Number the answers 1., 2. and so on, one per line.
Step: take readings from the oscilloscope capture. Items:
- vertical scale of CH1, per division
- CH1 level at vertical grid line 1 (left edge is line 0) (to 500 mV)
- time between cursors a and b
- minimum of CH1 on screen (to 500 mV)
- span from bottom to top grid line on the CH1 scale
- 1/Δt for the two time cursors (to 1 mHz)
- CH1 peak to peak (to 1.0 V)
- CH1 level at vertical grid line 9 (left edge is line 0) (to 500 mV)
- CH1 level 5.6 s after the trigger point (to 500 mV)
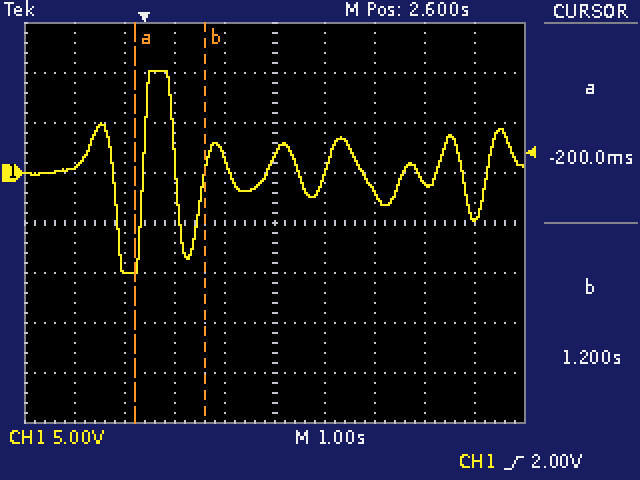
1. 5 V
2. 500 mV
3. 1.4 s
4. -10.0 V
5. 40 V
6. 714 mHz
7. 20.0 V
8. -4.5 V
9. -1.0 V
